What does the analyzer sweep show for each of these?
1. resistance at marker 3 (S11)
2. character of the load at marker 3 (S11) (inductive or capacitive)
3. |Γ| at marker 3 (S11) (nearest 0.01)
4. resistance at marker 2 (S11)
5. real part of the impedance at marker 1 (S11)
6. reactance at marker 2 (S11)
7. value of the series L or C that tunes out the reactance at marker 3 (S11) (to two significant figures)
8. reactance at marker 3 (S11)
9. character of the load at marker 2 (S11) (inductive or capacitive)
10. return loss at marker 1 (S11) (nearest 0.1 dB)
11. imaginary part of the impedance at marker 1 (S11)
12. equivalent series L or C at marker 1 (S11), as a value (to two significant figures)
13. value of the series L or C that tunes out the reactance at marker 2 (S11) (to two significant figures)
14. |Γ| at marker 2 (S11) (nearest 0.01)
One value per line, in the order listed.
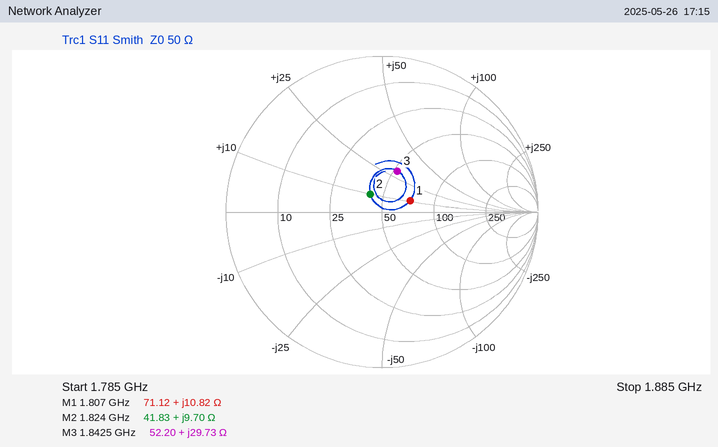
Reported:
52.20 Ω
inductive
0.28
41.83 Ω
71.12 Ω
+9.70 Ω
2.9 pF
+29.73 Ω
inductive
14.2 dB
+10.82 Ω
950 pH
9.0 pF
0.14
